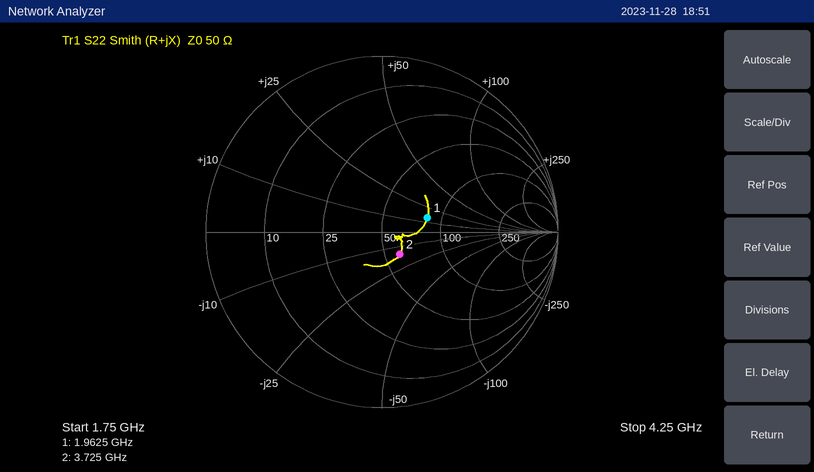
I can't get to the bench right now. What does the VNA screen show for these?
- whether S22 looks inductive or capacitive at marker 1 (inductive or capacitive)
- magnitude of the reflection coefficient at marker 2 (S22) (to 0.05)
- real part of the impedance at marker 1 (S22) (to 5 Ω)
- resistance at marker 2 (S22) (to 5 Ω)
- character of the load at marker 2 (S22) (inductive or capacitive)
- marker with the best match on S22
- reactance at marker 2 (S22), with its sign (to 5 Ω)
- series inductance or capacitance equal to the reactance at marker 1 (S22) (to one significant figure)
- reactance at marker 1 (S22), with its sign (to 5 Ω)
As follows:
inductive
0.15
85 Ω
60 Ω
capacitive
marker 2
-15 Ω
1 nH
+15 Ω
